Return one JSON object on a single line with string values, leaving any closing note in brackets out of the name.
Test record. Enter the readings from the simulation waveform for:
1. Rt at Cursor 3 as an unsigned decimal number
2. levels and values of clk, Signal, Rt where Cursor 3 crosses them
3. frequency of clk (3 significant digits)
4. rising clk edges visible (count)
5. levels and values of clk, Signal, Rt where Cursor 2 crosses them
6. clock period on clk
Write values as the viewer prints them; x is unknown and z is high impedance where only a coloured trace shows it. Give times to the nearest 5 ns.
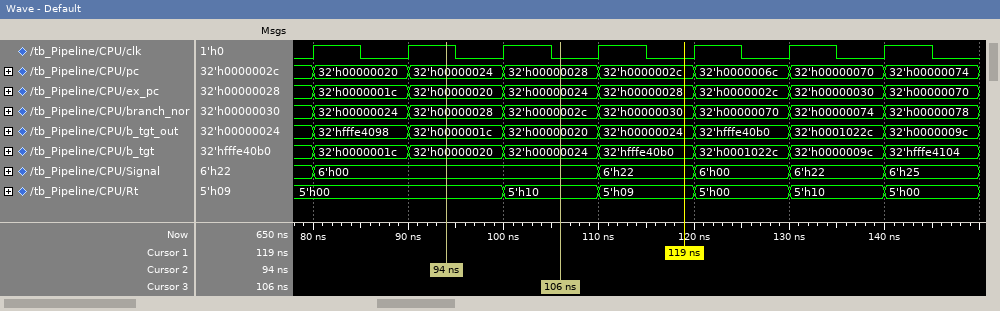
{"Rt at Cursor 3 as an unsigned decimal number": "16", "levels and values of clk, Signal, Rt where Cursor 3 crosses them": "clk=0, Signal=6'h00, Rt=5'h10", "frequency of clk": "100 MHz", "rising clk edges visible": "7", "levels and values of clk, Signal, Rt where Cursor 2 crosses them": "clk=1, Signal=6'h00, Rt=5'h00", "clock period on clk": "10 ns"}
